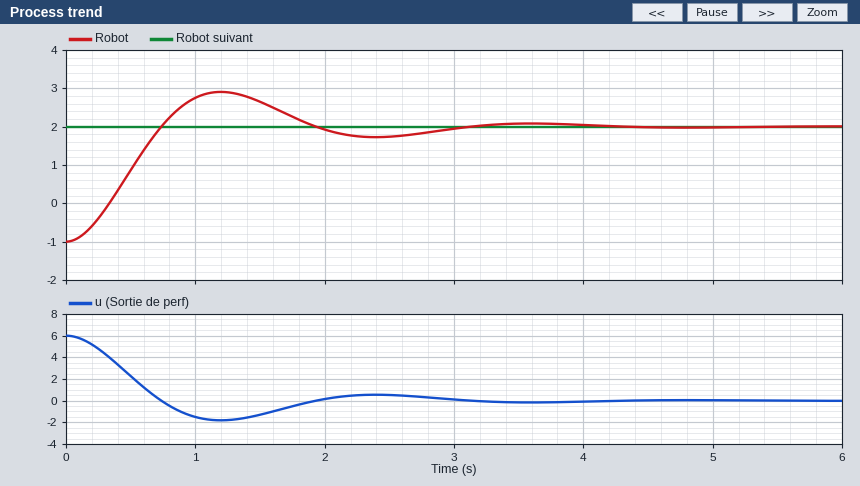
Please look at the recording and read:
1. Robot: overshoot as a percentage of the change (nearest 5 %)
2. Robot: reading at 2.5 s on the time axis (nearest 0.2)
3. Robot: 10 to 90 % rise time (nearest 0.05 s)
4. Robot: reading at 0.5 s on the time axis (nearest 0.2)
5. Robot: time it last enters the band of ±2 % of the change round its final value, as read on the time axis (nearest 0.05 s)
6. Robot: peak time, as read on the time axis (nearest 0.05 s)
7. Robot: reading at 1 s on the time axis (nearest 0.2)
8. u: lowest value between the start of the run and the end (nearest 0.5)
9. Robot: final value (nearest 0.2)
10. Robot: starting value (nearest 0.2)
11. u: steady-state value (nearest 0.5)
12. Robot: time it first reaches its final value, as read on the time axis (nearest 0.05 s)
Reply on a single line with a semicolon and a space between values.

30 %; 1.8; 0.50 s; 0.8; 3.90 s; 1.20 s; 2.8; -2.0; 2.0; -1.0; 0.0; 0.75 s
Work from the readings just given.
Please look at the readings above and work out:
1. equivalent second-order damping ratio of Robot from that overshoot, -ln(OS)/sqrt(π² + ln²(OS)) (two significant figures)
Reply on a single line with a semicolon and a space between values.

0.36
